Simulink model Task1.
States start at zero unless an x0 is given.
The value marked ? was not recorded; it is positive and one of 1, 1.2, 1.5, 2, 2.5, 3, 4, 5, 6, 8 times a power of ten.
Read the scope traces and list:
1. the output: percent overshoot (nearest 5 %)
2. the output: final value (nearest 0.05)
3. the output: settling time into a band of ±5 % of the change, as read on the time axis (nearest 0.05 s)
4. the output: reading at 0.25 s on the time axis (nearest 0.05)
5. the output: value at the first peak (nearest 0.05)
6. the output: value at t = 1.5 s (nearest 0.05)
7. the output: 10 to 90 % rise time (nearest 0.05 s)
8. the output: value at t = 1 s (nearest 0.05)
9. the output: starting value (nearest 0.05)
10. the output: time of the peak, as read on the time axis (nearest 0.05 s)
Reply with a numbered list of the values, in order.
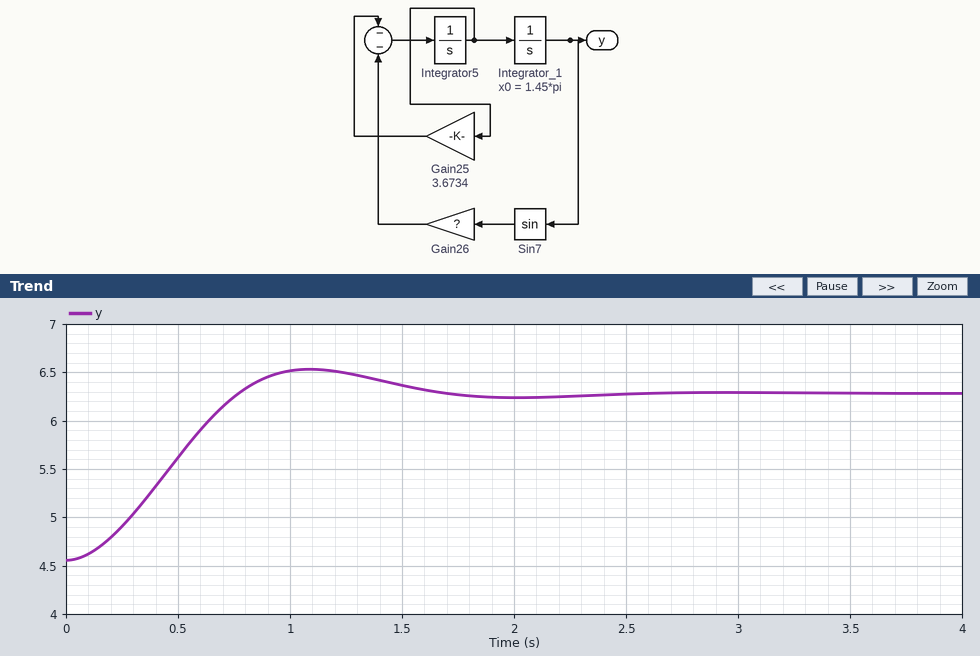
1. 15 %
2. 6.30
3. 1.50 s
4. 4.90
5. 6.55
6. 6.35
7. 0.50 s
8. 6.50
9. 4.55
10. 1.10 s
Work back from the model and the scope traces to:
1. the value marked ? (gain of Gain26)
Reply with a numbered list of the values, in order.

1. 15
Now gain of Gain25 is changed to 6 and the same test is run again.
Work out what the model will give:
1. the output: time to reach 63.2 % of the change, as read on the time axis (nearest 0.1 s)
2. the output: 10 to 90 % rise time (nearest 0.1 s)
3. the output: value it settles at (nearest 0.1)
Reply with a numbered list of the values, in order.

1. 0.6 s
2. 0.8 s
3. 6.3
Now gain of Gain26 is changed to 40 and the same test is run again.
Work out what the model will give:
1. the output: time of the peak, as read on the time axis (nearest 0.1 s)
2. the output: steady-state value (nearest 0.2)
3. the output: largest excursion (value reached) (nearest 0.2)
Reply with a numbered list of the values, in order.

1. 0.6 s
2. 6.2
3. 6.8
